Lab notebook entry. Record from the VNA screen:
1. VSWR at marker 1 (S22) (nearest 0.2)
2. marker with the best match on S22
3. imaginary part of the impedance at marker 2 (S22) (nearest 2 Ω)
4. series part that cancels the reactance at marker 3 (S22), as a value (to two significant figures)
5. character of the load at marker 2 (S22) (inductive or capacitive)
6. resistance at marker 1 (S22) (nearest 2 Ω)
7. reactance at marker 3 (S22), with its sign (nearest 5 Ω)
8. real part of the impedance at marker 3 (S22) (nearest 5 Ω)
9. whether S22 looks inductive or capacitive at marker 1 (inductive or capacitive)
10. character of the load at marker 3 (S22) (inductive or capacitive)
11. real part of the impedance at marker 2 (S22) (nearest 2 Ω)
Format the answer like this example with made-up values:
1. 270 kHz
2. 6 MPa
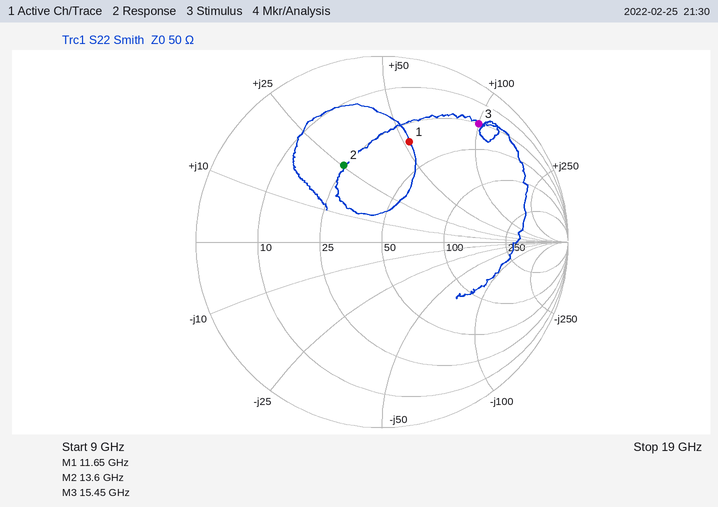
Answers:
1. 3.6
2. marker 2
3. +26 Ω
4. 100 fF
5. inductive
6. 34 Ω
7. +100 Ω
8. 25 Ω
9. inductive
10. inductive
11. 24 Ω
